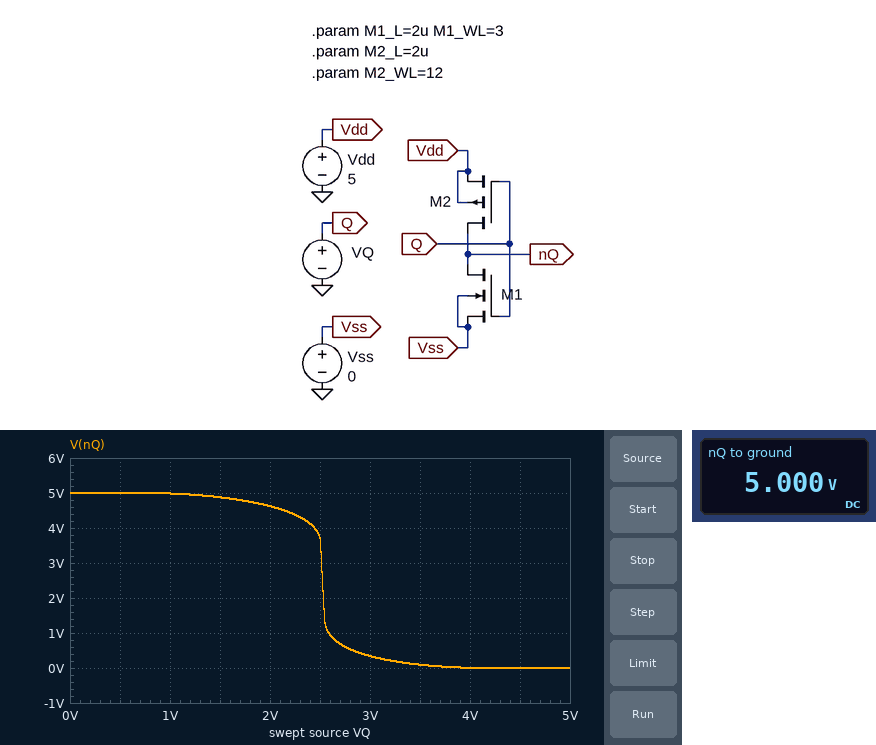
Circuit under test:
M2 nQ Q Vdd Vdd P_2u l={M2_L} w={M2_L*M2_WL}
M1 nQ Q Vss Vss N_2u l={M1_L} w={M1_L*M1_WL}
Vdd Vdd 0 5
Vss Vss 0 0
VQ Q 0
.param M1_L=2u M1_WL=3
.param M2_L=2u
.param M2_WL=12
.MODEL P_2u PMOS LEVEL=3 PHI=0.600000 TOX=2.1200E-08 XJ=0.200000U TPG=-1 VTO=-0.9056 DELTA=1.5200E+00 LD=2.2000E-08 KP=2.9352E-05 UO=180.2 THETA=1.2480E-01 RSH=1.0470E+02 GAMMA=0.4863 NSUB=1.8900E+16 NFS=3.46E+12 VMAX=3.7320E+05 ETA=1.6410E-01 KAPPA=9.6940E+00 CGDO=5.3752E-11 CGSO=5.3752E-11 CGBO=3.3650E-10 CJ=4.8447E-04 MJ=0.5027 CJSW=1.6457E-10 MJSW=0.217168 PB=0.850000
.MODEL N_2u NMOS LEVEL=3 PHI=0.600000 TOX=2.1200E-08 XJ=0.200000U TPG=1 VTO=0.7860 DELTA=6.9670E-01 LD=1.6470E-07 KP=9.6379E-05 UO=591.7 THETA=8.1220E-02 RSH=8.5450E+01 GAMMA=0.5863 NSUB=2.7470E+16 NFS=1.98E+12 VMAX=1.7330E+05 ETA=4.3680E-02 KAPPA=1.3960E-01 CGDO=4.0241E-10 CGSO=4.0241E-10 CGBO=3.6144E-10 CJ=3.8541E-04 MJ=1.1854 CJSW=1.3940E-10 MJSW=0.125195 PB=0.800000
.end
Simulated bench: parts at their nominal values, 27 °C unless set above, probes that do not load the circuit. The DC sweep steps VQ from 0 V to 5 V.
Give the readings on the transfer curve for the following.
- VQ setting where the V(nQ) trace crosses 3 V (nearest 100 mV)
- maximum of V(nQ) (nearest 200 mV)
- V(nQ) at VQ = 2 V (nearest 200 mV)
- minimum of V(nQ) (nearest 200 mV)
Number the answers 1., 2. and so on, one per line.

1. 2.5 V
2. 5.0 V
3. 4.6 V
4. 0 V
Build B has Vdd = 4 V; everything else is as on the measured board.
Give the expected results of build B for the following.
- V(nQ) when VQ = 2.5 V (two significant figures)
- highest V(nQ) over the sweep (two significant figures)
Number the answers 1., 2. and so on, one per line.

1. 130 mV
2. 4.0 V
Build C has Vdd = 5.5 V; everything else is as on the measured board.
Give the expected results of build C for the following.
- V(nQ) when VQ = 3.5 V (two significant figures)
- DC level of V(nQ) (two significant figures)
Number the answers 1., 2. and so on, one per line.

1. 290 mV
2. 5.5 V
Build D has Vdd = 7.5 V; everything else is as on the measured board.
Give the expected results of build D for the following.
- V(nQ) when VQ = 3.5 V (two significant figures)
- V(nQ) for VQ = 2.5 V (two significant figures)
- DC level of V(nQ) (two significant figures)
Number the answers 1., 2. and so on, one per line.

1. 6.2 V
2. 7.1 V
3. 7.5 V
